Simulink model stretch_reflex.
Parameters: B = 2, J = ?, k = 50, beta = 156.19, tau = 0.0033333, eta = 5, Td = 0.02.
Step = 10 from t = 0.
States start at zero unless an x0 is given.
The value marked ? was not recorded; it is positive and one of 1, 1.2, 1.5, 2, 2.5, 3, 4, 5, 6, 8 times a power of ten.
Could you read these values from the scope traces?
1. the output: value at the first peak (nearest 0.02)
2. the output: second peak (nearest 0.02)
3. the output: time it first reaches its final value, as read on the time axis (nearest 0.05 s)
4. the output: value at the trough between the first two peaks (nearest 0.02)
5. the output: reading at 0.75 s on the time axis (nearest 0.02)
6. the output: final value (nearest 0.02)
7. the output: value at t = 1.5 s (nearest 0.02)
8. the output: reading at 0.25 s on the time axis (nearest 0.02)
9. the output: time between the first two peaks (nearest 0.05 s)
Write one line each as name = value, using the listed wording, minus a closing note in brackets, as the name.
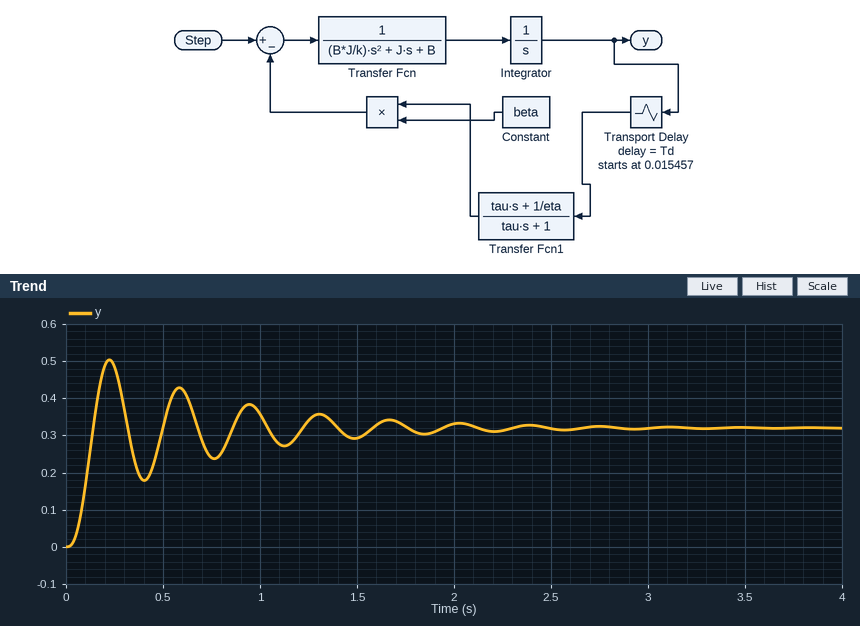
the output: value at the first peak = 0.50
the output: second peak = 0.42
the output: time it first reaches its final value, as read on the time axis = 0.15 s
the output: value at the trough between the first two peaks = 0.18
the output: reading at 0.75 s on the time axis = 0.24
the output: final value = 0.32
the output: value at t = 1.5 s = 0.30
the output: reading at 0.25 s on the time axis = 0.48
the output: time between the first two peaks = 0.35 s
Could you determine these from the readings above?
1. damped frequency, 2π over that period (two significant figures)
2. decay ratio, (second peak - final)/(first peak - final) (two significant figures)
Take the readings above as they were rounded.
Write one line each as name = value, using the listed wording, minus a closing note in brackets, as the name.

damped frequency, 2π over that period = 18 rad/s
decay ratio, (second peak - final)/(first peak - final) = 0.56
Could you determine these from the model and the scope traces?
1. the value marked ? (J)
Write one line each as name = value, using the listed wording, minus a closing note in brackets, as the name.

the value marked ? = 0.12
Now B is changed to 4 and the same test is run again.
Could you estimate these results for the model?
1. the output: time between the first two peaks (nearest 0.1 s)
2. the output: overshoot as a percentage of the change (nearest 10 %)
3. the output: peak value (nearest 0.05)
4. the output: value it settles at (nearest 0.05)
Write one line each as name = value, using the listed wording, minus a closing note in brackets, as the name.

the output: time between the first two peaks = 0.3 s
the output: overshoot as a percentage of the change = 20 %
the output: peak value = 0.40
the output: value it settles at = 0.30
